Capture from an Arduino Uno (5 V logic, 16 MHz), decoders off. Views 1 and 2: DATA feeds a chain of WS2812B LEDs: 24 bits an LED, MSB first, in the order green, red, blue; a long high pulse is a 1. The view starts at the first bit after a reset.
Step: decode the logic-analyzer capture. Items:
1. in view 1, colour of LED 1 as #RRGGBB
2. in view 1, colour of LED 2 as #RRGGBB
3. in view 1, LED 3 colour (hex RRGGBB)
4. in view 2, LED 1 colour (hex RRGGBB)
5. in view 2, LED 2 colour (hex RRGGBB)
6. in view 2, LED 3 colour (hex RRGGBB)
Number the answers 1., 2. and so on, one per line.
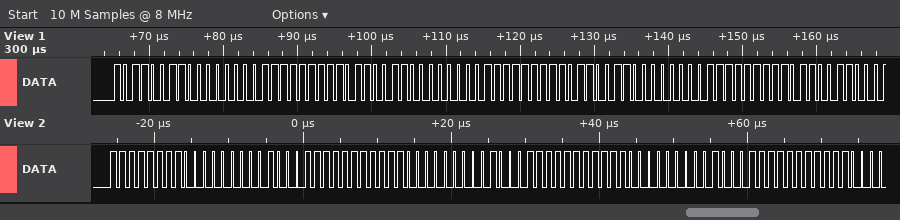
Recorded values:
1. #00B3FF
2. #00B3FF
3. #00B3FF
4. #00FF47
5. #00FF47
6. #00FF47
